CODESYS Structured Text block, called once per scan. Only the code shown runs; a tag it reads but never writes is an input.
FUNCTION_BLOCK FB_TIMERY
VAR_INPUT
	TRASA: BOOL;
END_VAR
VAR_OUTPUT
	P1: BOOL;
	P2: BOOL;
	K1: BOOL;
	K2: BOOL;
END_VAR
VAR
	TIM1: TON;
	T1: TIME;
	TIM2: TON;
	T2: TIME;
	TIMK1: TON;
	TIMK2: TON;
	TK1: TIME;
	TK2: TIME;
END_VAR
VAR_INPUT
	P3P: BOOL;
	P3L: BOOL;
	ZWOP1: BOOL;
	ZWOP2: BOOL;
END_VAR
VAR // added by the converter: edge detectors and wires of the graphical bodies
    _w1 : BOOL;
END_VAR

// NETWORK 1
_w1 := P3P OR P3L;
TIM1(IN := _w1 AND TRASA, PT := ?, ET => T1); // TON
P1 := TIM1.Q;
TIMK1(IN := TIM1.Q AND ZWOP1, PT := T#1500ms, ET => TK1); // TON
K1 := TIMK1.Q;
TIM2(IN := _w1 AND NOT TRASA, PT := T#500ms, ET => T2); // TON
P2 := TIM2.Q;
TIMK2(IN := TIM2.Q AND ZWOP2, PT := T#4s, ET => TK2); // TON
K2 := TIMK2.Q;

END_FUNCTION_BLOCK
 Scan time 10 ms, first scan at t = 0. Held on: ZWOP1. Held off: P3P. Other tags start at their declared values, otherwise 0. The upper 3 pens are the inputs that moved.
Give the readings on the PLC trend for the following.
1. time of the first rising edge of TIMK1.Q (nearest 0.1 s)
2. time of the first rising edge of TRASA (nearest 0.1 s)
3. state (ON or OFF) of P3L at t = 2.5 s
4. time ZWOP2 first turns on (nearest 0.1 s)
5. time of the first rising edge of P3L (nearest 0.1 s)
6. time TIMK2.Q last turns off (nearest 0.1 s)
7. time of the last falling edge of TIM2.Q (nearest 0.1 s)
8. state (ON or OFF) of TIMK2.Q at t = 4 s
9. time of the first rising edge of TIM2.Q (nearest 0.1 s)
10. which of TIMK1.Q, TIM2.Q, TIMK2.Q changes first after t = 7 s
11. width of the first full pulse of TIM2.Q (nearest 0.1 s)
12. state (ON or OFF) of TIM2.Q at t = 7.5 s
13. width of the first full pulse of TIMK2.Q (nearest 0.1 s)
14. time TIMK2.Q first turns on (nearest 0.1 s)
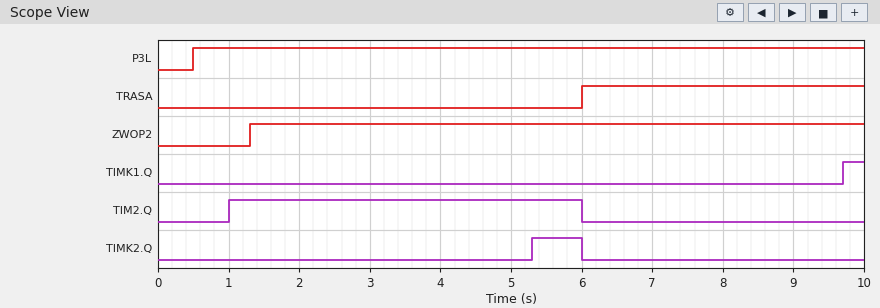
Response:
9.7 s
6.0 s
ON
1.3 s
0.5 s
6.0 s
6.0 s
OFF
1.0 s
TIMK1.Q
5.0 s
OFF
0.7 s
5.3 s
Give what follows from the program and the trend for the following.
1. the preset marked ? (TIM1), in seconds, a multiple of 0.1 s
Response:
2.2 s
